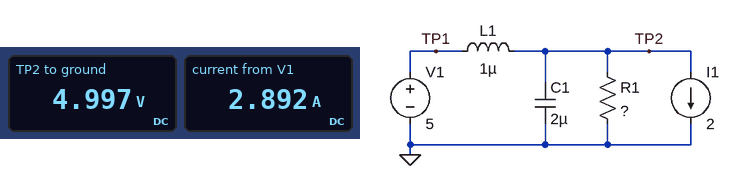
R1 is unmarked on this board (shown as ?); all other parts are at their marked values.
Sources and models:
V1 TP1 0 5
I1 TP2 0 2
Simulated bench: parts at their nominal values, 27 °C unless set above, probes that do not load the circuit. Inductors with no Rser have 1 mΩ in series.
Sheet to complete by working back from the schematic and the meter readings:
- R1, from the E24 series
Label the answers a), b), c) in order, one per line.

a) 5.6 Ω
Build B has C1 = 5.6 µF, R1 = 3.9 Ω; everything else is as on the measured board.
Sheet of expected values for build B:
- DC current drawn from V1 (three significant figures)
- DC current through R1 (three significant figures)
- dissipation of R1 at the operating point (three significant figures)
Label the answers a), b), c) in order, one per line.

a) 3.28 A
b) 1.28 A
c) 6.40 W
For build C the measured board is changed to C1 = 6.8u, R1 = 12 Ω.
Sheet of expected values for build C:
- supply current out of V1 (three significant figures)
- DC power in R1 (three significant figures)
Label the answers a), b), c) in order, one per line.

a) 2.42 A
b) 2.08 W
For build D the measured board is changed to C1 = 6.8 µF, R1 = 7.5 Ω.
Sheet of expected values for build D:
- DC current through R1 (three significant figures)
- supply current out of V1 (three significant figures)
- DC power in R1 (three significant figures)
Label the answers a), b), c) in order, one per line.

a) 666 mA
b) 2.67 A
c) 3.33 W
